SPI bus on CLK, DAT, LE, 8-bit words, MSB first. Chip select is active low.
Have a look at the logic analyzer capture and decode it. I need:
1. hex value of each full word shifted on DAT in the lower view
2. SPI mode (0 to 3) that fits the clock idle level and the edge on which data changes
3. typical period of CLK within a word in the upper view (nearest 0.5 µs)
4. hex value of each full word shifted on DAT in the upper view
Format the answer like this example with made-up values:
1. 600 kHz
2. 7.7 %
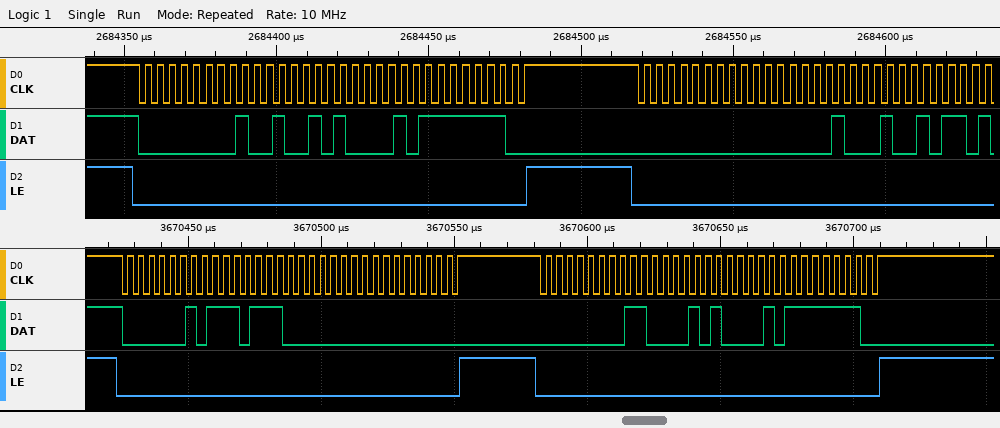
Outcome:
1. 02, EE, 00, 00, 00, C2, 85, FC
2. 3
3. 4 µs
4. 00, 92, 85, FC, 00, 00, 89
